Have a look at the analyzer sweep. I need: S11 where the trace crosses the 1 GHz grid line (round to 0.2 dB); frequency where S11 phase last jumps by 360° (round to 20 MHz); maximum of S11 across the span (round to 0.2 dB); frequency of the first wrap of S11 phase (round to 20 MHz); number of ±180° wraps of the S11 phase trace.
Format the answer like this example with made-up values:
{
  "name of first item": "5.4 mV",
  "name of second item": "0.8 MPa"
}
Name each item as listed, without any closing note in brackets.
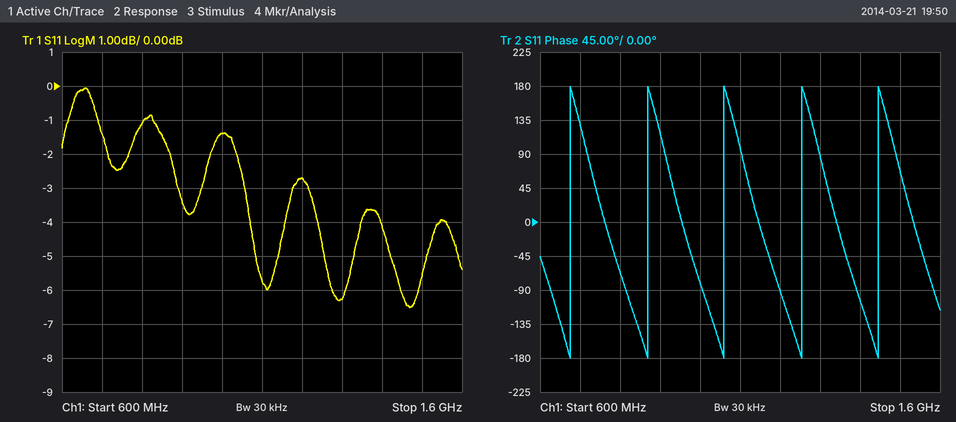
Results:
{
  "S11 where the trace crosses the 1 GHz grid line": "-1.4 dB",
  "frequency where S11 phase last jumps by 360°": "1.44 GHz",
  "maximum of S11 across the span": "0.0 dB",
  "frequency of the first wrap of S11 phase": "680 MHz",
  "number of ±180° wraps of the S11 phase trace": "5"
}
